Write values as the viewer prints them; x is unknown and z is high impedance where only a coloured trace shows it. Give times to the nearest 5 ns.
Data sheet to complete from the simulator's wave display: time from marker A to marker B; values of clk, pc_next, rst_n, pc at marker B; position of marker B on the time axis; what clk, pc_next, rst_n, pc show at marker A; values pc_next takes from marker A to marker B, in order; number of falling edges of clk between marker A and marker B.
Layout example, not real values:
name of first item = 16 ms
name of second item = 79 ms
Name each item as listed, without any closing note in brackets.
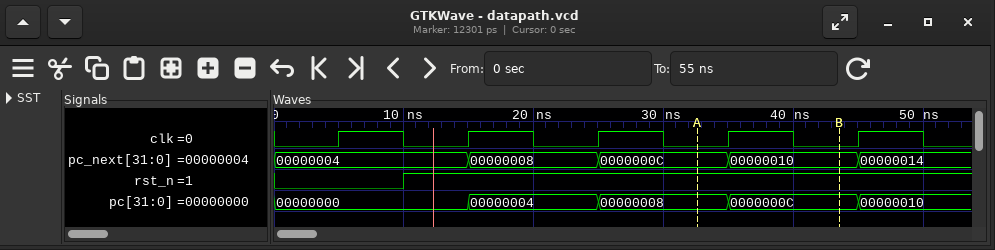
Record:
time from marker A to marker B = 10 ns
values of clk, pc_next, rst_n, pc at marker B = clk=0, pc_next=00000010, rst_n=1, pc=0000000C
position of marker B on the time axis = 45 ns
what clk, pc_next, rst_n, pc show at marker A = clk=0, pc_next=0000000C, rst_n=1, pc=00000008
values pc_next takes from marker A to marker B, in order = 0000000C, 00000010
number of falling edges of clk between marker A and marker B = 1
